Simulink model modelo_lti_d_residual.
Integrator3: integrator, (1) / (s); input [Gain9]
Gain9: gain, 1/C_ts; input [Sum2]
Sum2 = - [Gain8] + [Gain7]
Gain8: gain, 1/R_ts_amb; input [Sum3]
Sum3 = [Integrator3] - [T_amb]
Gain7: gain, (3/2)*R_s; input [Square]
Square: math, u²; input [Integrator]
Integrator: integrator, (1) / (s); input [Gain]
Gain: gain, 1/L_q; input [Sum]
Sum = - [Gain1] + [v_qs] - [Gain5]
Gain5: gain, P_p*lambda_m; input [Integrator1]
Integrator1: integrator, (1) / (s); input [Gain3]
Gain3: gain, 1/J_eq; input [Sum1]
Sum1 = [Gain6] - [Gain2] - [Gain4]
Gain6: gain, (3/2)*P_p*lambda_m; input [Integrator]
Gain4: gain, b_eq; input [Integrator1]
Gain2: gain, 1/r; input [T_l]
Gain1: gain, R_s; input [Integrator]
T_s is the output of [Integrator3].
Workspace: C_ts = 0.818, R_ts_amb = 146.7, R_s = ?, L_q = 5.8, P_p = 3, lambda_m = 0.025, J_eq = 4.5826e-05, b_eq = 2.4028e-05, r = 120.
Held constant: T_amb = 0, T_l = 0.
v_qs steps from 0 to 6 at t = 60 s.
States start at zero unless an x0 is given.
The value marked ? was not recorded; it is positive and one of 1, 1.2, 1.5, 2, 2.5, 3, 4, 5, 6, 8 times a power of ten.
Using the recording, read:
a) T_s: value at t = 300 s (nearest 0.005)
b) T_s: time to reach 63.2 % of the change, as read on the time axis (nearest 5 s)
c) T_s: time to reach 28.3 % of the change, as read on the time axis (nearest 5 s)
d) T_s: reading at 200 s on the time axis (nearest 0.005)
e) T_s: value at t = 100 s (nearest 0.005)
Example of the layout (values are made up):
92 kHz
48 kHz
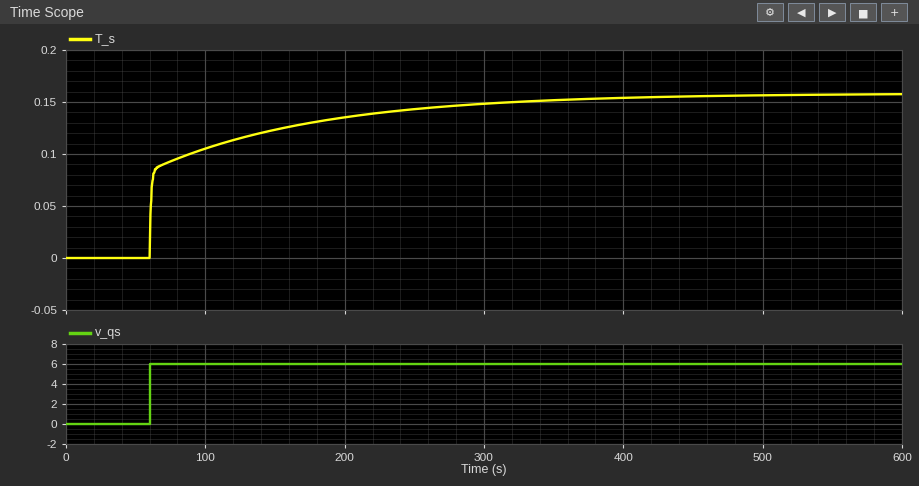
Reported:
0.150
90 s
60 s
0.135
0.105
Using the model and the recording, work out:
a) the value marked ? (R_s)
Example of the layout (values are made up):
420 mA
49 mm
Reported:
2.5
